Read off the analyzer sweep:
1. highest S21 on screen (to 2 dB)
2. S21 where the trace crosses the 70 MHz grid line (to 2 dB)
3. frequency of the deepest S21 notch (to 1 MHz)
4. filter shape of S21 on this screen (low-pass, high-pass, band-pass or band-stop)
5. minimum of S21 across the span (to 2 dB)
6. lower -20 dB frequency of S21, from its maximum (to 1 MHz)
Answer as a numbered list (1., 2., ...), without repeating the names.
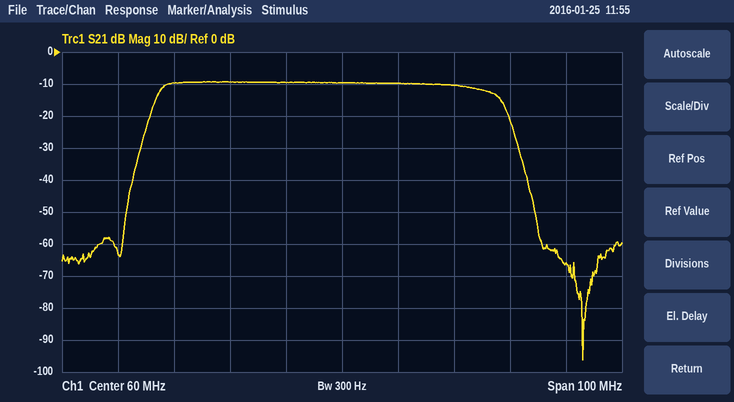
1. -10 dB
2. -10 dB
3. 103 MHz
4. band-pass
5. -96 dB
6. 24 MHz
